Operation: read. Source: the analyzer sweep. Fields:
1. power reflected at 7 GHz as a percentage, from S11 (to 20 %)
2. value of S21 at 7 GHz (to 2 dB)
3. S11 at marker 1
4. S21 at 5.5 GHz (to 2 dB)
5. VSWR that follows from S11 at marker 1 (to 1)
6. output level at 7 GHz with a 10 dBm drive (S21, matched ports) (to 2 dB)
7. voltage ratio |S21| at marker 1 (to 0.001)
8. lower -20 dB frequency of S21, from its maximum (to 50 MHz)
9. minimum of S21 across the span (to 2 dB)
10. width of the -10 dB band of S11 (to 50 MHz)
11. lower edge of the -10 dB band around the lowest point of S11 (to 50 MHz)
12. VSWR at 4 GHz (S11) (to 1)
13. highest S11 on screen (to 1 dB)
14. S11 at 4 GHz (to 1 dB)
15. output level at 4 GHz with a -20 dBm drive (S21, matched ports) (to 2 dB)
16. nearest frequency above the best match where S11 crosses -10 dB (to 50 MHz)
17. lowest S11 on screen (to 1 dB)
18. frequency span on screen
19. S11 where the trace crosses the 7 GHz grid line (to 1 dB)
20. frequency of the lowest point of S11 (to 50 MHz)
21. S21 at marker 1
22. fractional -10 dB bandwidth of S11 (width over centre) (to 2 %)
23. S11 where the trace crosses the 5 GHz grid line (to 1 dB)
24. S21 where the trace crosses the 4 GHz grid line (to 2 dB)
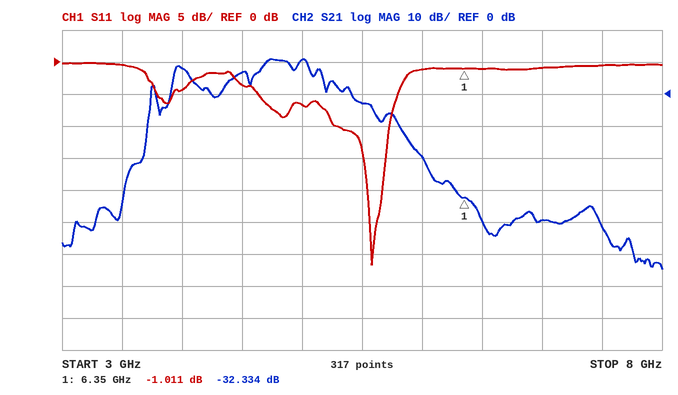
80 %
-40 dB
-1.011 dB
-2 dB
17
-30 dBm
0.024
3.70 GHz
-54 dB
450 MHz
5.30 GHz
4
0 dB
-4 dB
-12 dBm
5.75 GHz
-32 dB
5 GHz
-1 dB
5.60 GHz
-32.334 dB
8 %
-7 dB
8 dB
